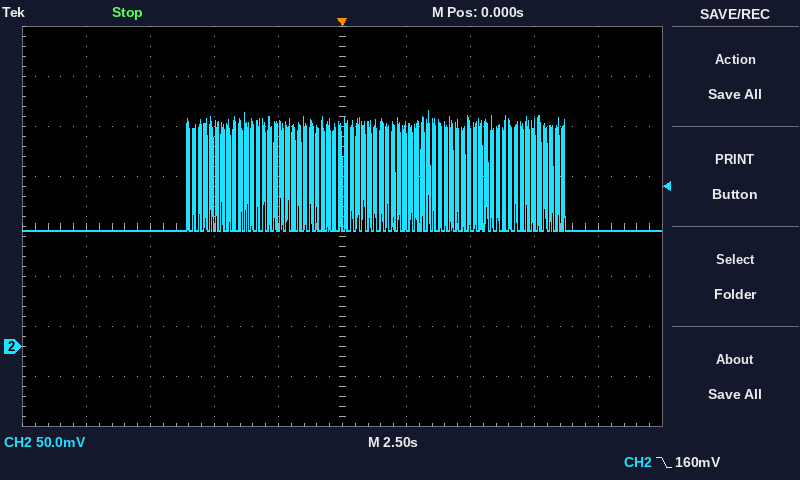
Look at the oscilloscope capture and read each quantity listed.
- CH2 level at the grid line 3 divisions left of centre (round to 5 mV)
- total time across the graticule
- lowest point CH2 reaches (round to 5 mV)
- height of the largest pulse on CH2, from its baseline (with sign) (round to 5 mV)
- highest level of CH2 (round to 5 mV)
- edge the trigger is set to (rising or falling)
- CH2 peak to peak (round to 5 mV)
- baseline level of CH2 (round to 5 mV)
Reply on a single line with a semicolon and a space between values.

115 mV; 25 s; 115 mV; +120 mV; 235 mV; falling; 120 mV; 115 mV
